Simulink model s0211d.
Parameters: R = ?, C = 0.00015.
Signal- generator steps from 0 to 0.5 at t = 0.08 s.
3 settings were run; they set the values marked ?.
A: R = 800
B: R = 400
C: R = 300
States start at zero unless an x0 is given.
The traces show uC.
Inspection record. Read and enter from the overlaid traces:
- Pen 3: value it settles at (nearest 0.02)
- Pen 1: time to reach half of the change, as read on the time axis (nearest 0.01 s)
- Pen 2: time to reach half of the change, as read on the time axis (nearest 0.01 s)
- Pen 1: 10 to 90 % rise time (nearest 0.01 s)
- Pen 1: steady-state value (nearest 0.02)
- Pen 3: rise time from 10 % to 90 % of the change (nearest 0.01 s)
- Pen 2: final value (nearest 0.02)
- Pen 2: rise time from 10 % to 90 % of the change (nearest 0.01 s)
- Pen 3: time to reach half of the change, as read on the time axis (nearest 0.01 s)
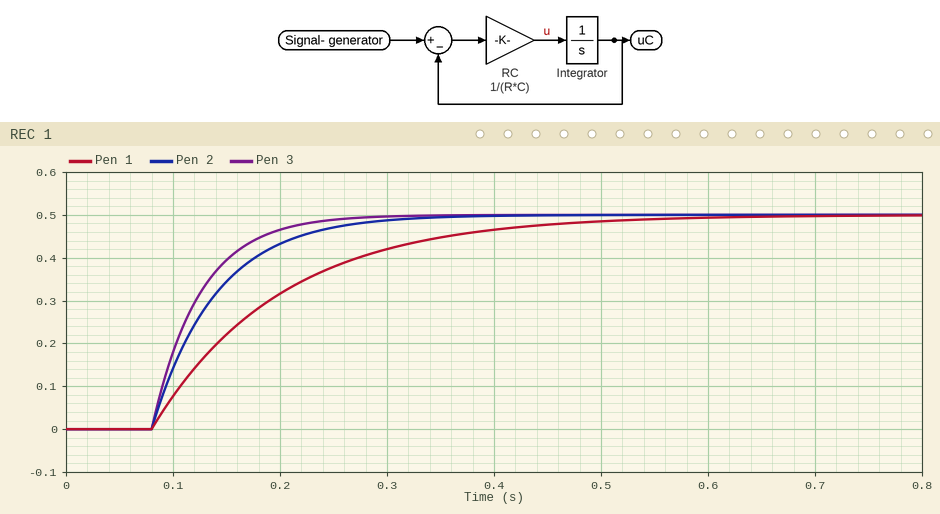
0.50
0.16 s
0.12 s
0.26 s
0.50
0.10 s
0.50
0.13 s
0.11 s
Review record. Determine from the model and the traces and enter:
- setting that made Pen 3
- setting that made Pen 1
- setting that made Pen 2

C
A
B
